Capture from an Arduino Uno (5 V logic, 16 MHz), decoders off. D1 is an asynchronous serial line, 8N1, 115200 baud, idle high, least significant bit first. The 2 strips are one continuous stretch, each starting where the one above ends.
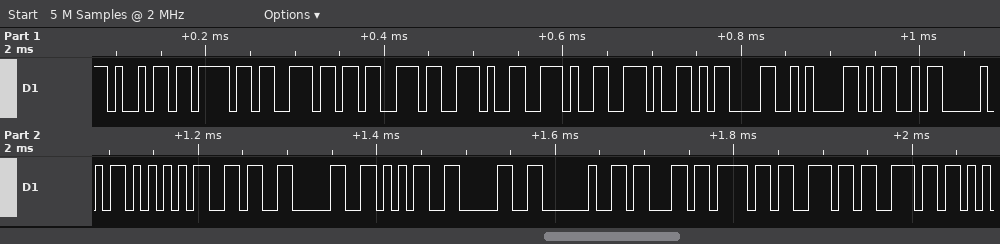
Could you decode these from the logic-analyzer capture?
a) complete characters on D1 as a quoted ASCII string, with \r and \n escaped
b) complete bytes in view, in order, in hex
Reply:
"ions...\r\nMPU6050 conn"
69 6F 6E 73 2E 2E 2E 0D 0A 4D 50 55 36 30 35 30 20 63 6F 6E 6E
